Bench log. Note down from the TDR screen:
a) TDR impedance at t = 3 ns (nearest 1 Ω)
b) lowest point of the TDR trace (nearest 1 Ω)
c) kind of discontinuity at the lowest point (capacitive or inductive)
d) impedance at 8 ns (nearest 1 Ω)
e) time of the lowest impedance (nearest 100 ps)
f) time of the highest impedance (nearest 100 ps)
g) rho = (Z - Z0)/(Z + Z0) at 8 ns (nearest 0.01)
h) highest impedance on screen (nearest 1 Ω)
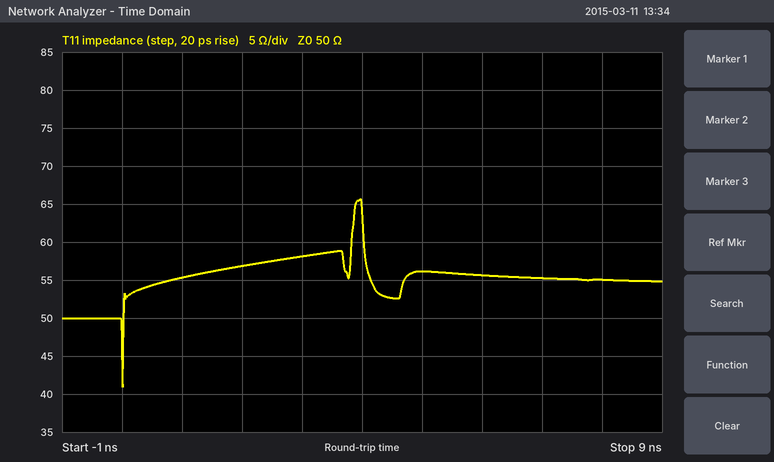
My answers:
58 Ω
41 Ω
capacitive
55 Ω
0.0 ns
4.0 ns
+0.05
66 Ω
